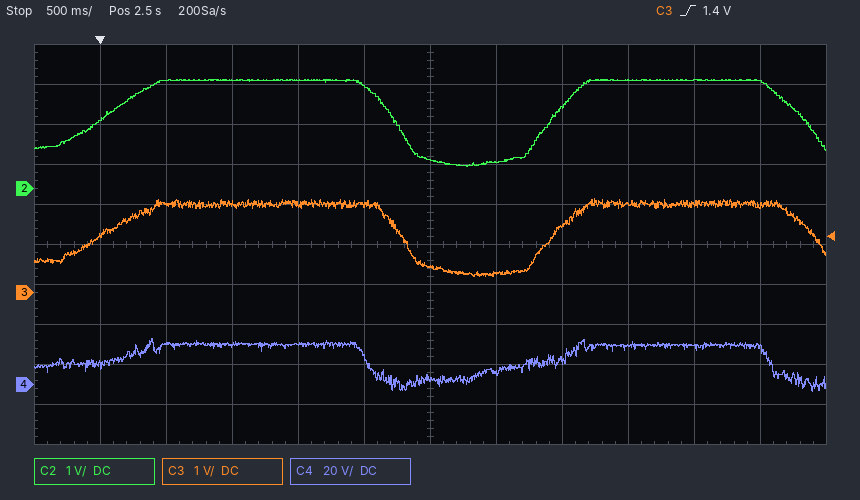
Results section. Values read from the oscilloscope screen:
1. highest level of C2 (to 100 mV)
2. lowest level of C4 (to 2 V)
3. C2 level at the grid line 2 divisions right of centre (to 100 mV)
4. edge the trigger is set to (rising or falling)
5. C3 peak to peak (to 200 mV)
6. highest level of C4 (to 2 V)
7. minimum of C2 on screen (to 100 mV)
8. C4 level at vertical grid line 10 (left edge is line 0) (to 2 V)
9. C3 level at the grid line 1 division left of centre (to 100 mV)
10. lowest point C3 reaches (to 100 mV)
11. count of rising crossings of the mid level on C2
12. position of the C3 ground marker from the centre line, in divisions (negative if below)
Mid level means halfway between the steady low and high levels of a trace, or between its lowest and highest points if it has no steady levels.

2.7 V
-4 V
2.0 V
rising
2.0 V
24 V
600 mV
18 V
2.2 V
400 mV
2
-1.2 div
